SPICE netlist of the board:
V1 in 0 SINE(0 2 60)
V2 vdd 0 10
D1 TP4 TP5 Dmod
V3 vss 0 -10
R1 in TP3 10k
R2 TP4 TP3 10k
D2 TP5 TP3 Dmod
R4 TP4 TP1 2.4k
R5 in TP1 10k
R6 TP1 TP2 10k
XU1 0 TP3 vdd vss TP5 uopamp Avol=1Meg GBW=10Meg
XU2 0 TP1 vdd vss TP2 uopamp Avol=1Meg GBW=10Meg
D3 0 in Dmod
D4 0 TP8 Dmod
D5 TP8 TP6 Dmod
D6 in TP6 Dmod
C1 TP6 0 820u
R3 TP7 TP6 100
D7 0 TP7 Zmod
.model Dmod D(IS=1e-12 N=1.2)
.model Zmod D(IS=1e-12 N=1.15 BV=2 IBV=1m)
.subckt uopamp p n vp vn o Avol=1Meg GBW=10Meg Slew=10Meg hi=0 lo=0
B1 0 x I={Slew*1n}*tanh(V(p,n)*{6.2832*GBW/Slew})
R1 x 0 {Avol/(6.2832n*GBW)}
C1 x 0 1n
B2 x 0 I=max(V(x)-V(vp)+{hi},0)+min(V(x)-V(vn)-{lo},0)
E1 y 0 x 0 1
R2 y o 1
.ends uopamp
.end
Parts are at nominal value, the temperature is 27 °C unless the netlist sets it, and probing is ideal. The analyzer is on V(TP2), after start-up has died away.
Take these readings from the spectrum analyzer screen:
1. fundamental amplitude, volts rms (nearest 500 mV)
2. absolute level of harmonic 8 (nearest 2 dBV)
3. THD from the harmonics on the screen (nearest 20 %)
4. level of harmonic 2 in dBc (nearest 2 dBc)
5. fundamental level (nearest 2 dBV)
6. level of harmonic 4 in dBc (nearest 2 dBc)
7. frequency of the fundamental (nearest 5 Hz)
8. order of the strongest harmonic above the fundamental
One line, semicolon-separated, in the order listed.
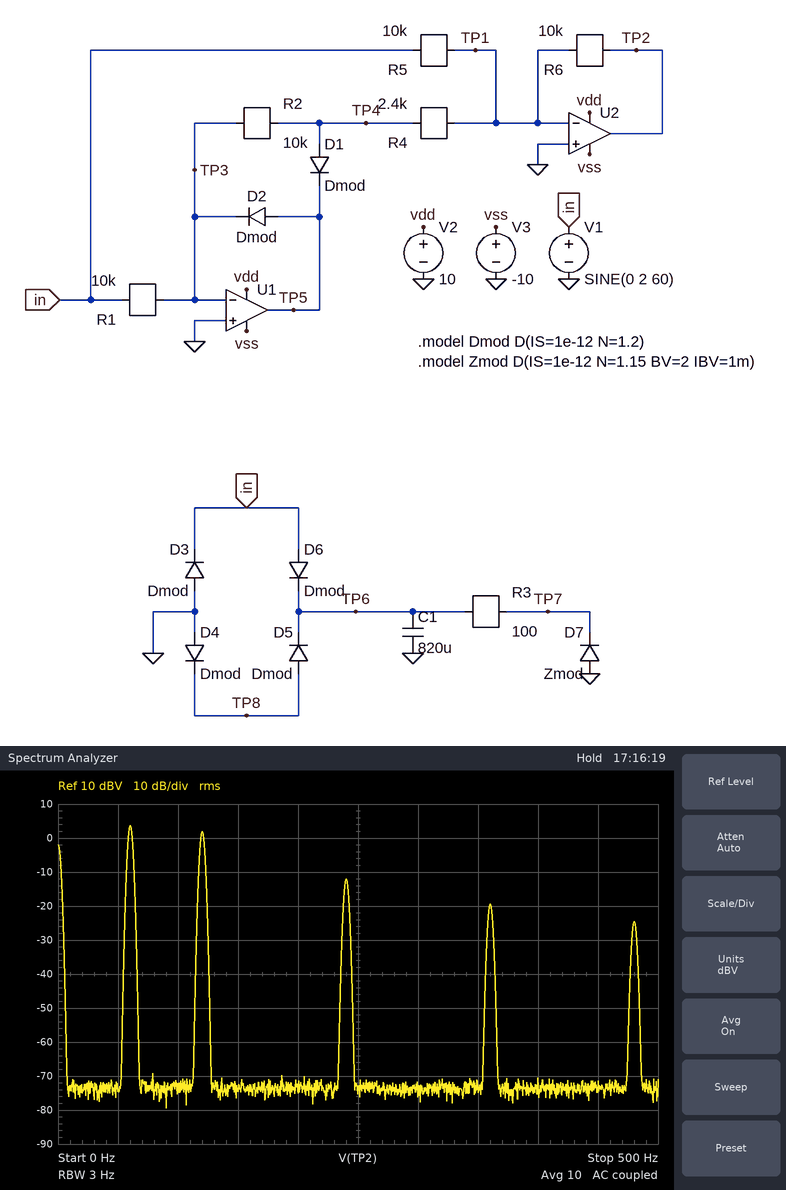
1.5 V; -24 dBV; 80 %; -2 dBc; 4 dBV; -16 dBc; 60 Hz; 2
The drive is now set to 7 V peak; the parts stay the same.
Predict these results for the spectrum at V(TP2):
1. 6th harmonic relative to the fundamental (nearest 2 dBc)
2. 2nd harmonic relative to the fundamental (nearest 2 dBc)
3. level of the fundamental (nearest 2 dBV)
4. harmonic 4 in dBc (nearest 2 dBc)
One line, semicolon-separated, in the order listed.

-10 dBc; 0 dBc; 6 dBV; -6 dBc
